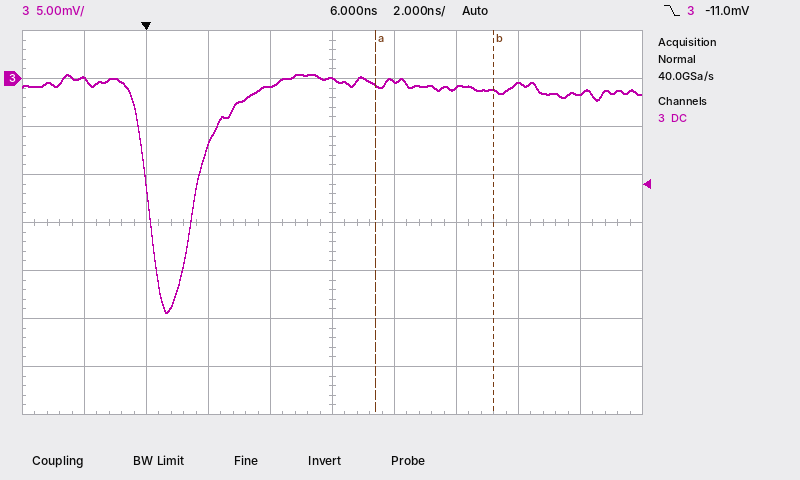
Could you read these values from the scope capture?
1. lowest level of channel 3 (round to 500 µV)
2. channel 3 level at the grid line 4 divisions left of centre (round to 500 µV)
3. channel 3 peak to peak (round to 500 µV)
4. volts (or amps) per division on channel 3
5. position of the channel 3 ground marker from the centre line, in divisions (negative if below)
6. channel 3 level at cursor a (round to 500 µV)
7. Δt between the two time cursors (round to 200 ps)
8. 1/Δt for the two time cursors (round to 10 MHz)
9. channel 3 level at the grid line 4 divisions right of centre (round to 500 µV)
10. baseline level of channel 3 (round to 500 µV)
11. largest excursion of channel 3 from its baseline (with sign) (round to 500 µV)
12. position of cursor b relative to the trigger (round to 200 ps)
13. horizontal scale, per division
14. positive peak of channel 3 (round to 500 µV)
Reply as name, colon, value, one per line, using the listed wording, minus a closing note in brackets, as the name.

lowest level of channel 3: -24.5 mV
channel 3 level at the grid line 4 divisions left of centre: 0.0 mV
channel 3 peak to peak: 25.0 mV
volts (or amps) per division on channel 3: 5 mV
position of the channel 3 ground marker from the centre line, in divisions: +3.0 div
channel 3 level at cursor a: -500 µV
Δt between the two time cursors: 3.8 ns
1/Δt for the two time cursors: 260 MHz
channel 3 level at the grid line 4 divisions right of centre: -1.5 mV
baseline level of channel 3: -1.0 mV
largest excursion of channel 3 from its baseline (with sign): -23.5 mV
position of cursor b relative to the trigger: +11.2 ns
horizontal scale, per division: 2 ns
positive peak of channel 3: 500 µV
